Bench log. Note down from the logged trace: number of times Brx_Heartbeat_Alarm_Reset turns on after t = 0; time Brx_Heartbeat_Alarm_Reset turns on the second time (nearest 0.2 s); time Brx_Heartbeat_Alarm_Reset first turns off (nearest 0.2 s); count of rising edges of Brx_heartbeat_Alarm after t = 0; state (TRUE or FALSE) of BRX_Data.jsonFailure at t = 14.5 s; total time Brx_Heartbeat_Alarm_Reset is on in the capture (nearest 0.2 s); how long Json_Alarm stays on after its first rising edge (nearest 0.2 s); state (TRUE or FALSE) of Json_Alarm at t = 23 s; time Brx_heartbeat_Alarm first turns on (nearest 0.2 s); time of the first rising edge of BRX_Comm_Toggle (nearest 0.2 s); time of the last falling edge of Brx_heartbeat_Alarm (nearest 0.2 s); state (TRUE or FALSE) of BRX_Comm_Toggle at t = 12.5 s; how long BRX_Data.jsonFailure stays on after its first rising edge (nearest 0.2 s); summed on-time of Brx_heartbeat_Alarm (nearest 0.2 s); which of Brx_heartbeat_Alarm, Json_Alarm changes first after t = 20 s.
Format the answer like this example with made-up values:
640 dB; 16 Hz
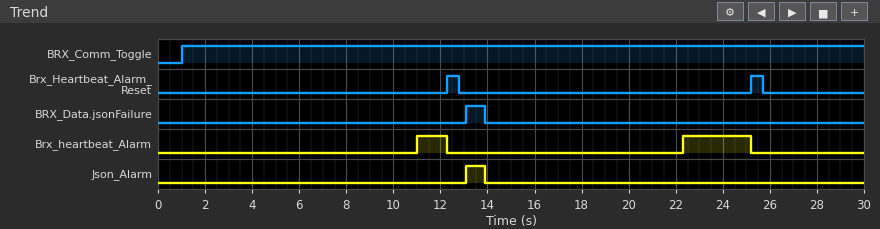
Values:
2; 25.2 s; 12.8 s; 2; FALSE; 1.0 s; 0.8 s; FALSE; 11.0 s; 1.0 s; 25.2 s; TRUE; 0.8 s; 4.2 s; Brx_heartbeat_Alarm
